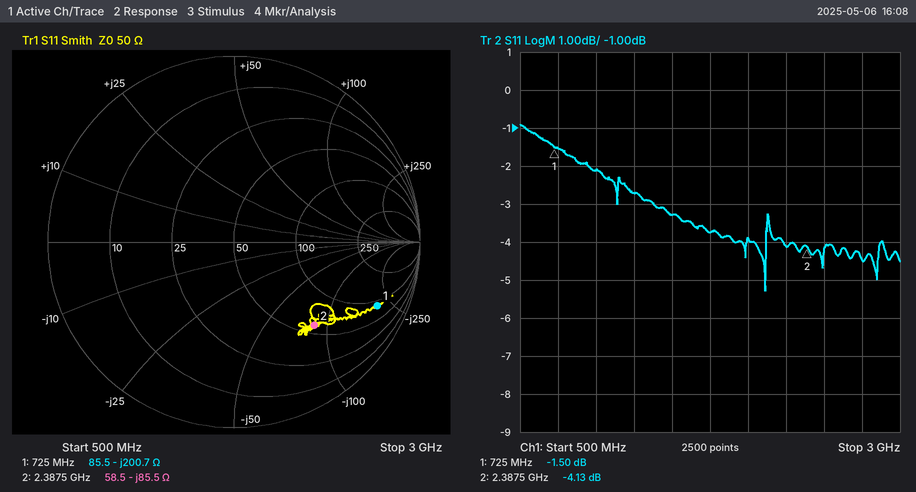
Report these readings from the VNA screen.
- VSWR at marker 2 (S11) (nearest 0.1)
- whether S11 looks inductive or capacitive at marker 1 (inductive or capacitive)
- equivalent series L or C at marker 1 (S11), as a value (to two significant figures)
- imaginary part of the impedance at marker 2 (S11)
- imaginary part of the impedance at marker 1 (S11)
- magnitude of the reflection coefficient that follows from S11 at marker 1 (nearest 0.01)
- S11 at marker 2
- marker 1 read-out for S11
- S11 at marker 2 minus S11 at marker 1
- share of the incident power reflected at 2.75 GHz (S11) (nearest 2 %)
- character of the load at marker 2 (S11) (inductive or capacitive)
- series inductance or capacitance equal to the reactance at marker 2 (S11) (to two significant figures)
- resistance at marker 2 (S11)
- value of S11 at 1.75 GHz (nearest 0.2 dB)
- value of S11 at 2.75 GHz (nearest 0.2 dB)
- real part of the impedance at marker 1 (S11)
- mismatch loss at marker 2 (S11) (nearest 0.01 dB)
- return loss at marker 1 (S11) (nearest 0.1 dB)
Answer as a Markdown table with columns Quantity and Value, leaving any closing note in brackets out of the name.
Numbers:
| Quantity | Value |
|---|---|
| VSWR at marker 2 (S11) | 4.3 |
| whether S11 looks inductive or capacitive at marker 1 | capacitive |
| equivalent series L or C at marker 1 (S11), as a value | 1.1 pF |
| imaginary part of the impedance at marker 2 | -85.5 Ω |
| imaginary part of the impedance at marker 1 | -200.7 Ω |
| magnitude of the reflection coefficient that follows from S11 at marker 1 | 0.84 |
| S11 at marker 2 | -4.13 dB |
| marker 1 read-out for S11 | -1.50 dB |
| S11 at marker 2 minus S11 at marker 1 | -2.63 dB |
| share of the incident power reflected at 2.75 GHz (S11) | 36 % |
| character of the load at marker 2 (S11) | capacitive |
| series inductance or capacitance equal to the reactance at marker 2 (S11) | 780 fF |
| resistance at marker 2 | 58.5 Ω |
| value of S11 at 1.75 GHz | -3.8 dB |
| value of S11 at 2.75 GHz | -4.4 dB |
| real part of the impedance at marker 1 | 85.5 Ω |
| mismatch loss at marker 2 (S11) | 2.12 dB |
| return loss at marker 1 (S11) | 1.5 dB |
